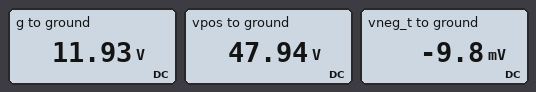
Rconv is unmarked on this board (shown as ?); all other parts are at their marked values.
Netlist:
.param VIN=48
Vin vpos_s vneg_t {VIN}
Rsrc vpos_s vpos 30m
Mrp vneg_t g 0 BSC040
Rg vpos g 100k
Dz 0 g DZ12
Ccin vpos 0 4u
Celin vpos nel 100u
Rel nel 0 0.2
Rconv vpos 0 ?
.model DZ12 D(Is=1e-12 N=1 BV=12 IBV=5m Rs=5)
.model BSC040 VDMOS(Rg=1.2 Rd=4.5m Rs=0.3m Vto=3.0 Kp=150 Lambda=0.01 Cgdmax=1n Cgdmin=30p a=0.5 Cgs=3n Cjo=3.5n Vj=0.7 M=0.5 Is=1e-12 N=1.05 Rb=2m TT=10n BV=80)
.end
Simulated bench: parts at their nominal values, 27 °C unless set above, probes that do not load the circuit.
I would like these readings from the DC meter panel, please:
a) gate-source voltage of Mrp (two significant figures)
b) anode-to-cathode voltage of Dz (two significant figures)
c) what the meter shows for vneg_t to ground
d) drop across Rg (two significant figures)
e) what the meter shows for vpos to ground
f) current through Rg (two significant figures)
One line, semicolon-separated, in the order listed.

12 V; -12 V; -9.8 mV; 36 V; 47.94 V; 360 µA
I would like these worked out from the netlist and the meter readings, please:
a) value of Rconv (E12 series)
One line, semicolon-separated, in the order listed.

27 Ω
